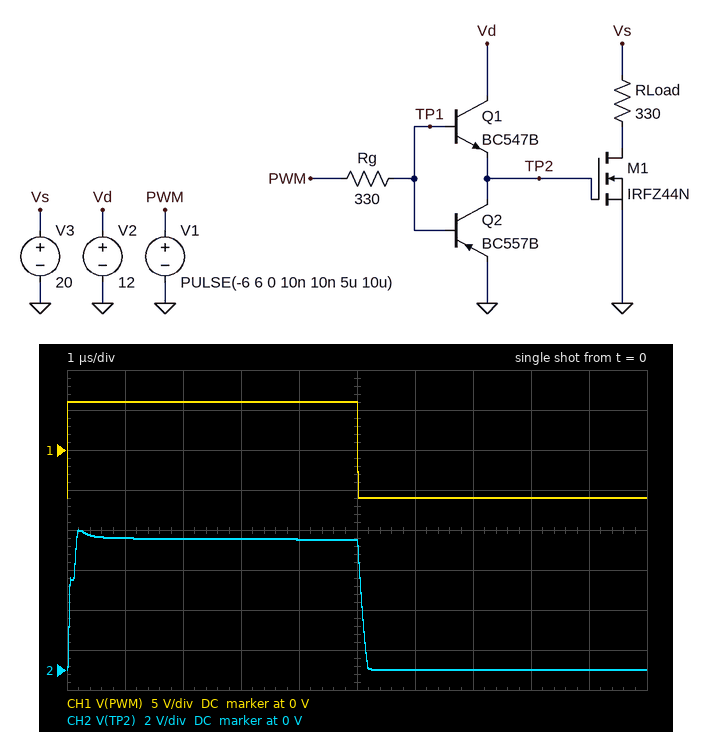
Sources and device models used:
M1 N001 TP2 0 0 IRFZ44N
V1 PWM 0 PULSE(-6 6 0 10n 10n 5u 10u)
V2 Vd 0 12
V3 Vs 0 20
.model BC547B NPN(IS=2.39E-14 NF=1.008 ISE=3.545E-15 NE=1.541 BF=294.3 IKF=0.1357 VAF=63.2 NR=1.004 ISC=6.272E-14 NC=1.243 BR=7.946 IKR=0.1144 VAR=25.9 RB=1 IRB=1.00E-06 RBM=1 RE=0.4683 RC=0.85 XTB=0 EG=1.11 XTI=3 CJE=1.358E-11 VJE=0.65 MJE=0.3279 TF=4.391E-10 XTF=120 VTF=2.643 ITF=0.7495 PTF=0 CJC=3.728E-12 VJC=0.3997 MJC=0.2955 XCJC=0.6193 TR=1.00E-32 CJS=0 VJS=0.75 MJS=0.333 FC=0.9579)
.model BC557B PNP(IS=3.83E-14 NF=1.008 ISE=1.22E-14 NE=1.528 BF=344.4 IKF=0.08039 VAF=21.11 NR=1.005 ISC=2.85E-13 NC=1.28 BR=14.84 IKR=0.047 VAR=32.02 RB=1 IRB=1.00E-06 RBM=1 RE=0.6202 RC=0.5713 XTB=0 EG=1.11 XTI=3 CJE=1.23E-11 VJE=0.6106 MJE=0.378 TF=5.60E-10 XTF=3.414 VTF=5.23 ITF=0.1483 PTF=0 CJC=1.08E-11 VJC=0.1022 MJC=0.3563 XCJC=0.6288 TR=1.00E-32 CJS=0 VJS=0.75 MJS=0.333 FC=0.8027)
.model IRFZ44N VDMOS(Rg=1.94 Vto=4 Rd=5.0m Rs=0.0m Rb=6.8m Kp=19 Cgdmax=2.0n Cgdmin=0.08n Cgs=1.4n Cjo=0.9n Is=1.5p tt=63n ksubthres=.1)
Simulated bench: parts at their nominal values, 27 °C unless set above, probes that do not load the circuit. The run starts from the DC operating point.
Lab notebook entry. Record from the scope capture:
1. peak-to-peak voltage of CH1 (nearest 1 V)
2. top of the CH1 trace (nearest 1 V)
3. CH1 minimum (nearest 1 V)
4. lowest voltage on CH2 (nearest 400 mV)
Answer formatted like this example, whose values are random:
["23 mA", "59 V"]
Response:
["12 V", "6 V", "-6 V", "0 V"]
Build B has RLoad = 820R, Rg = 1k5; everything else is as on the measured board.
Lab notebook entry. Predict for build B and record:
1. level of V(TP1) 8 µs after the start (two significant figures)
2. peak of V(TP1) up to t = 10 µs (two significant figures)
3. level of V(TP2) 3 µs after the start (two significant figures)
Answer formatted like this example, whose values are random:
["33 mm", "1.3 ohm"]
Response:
["-730 mV", "7.0 V", "6.3 V"]
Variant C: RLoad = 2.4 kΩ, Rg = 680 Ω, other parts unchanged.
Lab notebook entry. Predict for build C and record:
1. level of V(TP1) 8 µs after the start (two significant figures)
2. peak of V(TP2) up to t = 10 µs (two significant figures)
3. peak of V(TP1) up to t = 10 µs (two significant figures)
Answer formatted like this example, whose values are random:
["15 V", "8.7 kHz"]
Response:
["-760 mV", "6.8 V", "7.5 V"]
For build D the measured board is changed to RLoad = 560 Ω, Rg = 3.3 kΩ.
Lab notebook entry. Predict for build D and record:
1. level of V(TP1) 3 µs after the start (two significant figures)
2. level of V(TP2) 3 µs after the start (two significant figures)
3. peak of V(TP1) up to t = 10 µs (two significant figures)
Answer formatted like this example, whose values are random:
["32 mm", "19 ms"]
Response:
["6.0 V", "5.9 V", "6.6 V"]
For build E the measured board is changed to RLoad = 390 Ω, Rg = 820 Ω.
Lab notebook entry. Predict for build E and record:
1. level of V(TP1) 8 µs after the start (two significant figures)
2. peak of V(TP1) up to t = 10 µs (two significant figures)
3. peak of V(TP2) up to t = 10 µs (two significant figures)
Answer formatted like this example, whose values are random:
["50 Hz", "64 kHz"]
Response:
["-750 mV", "7.4 V", "6.7 V"]
